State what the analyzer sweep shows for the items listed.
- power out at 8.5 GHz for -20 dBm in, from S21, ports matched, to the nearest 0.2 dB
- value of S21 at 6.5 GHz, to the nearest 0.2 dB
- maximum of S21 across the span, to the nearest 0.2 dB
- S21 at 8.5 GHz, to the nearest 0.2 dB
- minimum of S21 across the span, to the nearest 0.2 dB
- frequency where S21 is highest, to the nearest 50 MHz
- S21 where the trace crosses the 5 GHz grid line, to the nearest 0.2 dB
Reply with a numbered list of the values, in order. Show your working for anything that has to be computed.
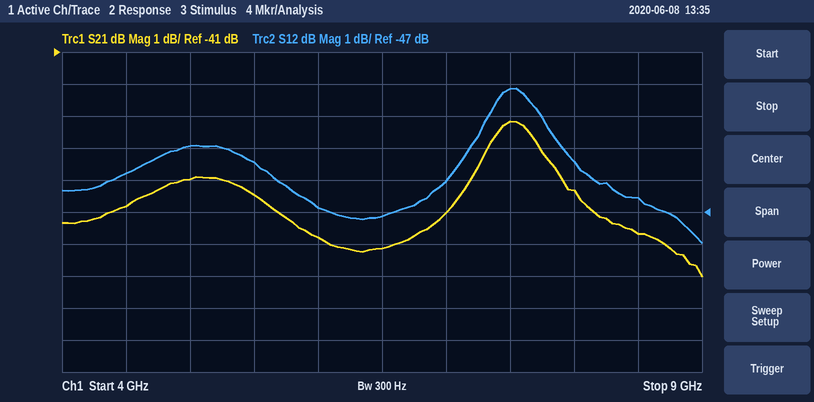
1. -20 dBm + (-46.6 dB) = -66.6 dBm
2. -47.2 dB
3. -43.2 dB
4. -46.6 dB
5. -48.0 dB
6. 7.50 GHz
7. -45.0 dB
